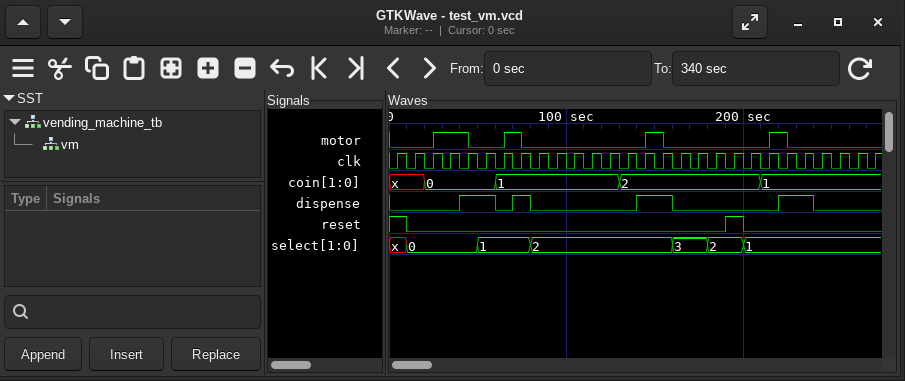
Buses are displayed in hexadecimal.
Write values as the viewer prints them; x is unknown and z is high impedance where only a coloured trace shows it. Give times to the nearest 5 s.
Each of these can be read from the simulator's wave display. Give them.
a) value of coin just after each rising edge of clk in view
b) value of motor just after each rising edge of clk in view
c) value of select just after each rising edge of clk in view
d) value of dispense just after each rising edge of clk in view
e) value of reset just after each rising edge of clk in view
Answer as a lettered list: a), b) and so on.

a) x, x, 0, 0, 0, 0, 1, 1, 1, 1, 1, 1, 1, 2, 2, 2, 2, 2, 2, 2, 2, 1, 1, 1, 1, 1, 1, 1
b) 0 0 1 1 0 0 1 0 0 0 0 0 0 0 1 0 0 0 0 0 0 1 0 0 0 0 0 0
c) x, 0, 0, 0, 0, 1, 1, 1, 2, 2, 2, 2, 2, 2, 2, 2, 3, 3, 2, 2, 1, 1, 1, 1, 1, 1, 1, 1
d) 0 0 0 0 1 1 0 1 0 0 0 0 0 0 1 1 0 0 0 0 0 0 1 1 0 0 0 0
e) 1 0 0 0 0 0 0 0 0 0 0 0 0 0 0 0 0 0 0 1 0 0 0 0 0 0 0 0
